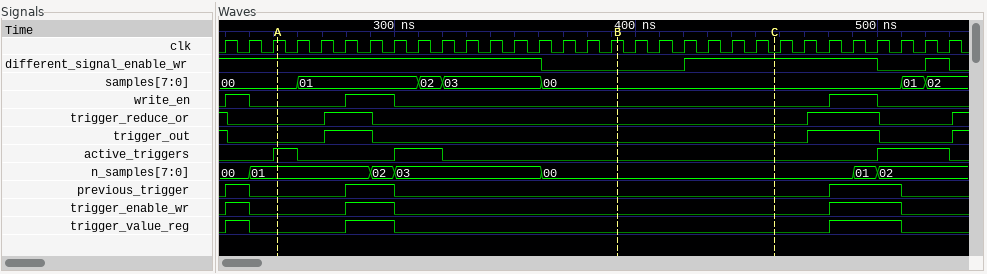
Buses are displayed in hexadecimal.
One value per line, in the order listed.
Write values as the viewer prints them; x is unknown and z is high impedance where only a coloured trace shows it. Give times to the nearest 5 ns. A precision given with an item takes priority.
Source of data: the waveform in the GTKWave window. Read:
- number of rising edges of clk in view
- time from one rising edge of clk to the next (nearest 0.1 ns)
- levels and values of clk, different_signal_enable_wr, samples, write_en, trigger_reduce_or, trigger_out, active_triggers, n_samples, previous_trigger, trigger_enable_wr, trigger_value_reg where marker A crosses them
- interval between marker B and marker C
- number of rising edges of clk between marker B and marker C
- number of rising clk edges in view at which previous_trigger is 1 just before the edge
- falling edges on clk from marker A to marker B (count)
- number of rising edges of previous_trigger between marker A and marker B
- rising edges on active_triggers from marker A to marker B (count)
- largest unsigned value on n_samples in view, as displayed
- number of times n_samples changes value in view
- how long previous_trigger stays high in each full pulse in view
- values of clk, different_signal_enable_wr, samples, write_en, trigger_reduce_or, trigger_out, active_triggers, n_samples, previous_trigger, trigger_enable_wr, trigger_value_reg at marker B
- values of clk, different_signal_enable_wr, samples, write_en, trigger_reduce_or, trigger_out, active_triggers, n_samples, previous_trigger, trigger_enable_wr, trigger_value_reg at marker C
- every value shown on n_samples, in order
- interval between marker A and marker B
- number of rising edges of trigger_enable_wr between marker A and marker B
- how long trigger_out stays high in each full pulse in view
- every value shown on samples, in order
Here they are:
31
10 ns
clk=1, different_signal_enable_wr=1, samples=00, write_en=0, trigger_reduce_or=0, trigger_out=0, active_triggers=1, n_samples=01, previous_trigger=0, trigger_enable_wr=0, trigger_value_reg=0
65 ns
6
6
14
1
1
03
6
10 ns, 20 ns, 30 ns
clk=1, different_signal_enable_wr=0, samples=00, write_en=0, trigger_reduce_or=0, trigger_out=0, active_triggers=0, n_samples=00, previous_trigger=0, trigger_enable_wr=0, trigger_value_reg=0
clk=0, different_signal_enable_wr=1, samples=00, write_en=0, trigger_reduce_or=0, trigger_out=0, active_triggers=0, n_samples=00, previous_trigger=0, trigger_enable_wr=0, trigger_value_reg=0
00, 01, 02, 03, 00, 01, 02
140 ns
1
20 ns, 30 ns
00, 01, 02, 03, 00, 01, 02
